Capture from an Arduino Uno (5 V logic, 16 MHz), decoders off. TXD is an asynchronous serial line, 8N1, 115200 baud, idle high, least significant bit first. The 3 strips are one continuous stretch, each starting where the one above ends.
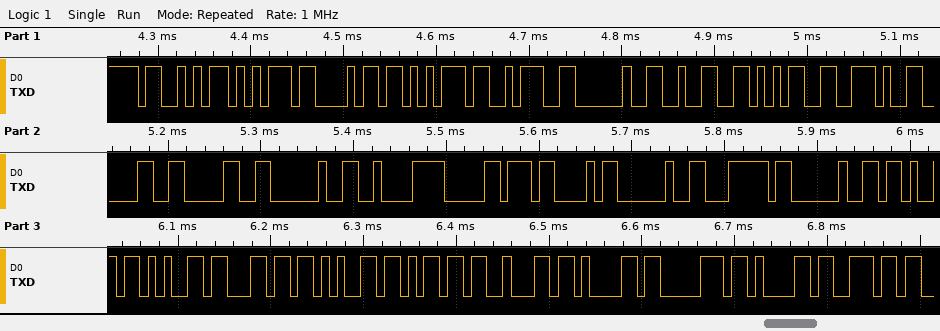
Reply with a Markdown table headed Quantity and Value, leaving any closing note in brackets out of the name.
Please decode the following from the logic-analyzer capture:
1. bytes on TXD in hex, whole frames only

| Quantity | Value |
|---|---|
| bytes on TXD in hex, whole frames only | 53 75 68 75 3A 20 32 35 2E 30 30 20 C2 B0 43 20 7C 20 4B 65 6C 65 6D 62 61 70 61 6E |
